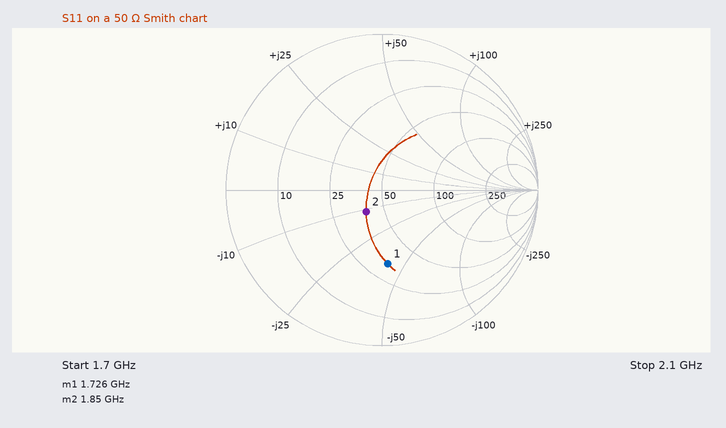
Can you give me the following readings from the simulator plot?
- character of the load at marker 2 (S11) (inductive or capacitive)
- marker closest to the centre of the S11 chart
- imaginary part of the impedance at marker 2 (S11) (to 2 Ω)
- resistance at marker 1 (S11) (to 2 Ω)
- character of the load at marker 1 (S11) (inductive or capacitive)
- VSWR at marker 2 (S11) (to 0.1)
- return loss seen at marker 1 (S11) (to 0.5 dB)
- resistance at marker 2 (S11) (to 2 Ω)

capacitive
marker 2
-12 Ω
34 Ω
capacitive
1.4
6.5 dB
40 Ω
